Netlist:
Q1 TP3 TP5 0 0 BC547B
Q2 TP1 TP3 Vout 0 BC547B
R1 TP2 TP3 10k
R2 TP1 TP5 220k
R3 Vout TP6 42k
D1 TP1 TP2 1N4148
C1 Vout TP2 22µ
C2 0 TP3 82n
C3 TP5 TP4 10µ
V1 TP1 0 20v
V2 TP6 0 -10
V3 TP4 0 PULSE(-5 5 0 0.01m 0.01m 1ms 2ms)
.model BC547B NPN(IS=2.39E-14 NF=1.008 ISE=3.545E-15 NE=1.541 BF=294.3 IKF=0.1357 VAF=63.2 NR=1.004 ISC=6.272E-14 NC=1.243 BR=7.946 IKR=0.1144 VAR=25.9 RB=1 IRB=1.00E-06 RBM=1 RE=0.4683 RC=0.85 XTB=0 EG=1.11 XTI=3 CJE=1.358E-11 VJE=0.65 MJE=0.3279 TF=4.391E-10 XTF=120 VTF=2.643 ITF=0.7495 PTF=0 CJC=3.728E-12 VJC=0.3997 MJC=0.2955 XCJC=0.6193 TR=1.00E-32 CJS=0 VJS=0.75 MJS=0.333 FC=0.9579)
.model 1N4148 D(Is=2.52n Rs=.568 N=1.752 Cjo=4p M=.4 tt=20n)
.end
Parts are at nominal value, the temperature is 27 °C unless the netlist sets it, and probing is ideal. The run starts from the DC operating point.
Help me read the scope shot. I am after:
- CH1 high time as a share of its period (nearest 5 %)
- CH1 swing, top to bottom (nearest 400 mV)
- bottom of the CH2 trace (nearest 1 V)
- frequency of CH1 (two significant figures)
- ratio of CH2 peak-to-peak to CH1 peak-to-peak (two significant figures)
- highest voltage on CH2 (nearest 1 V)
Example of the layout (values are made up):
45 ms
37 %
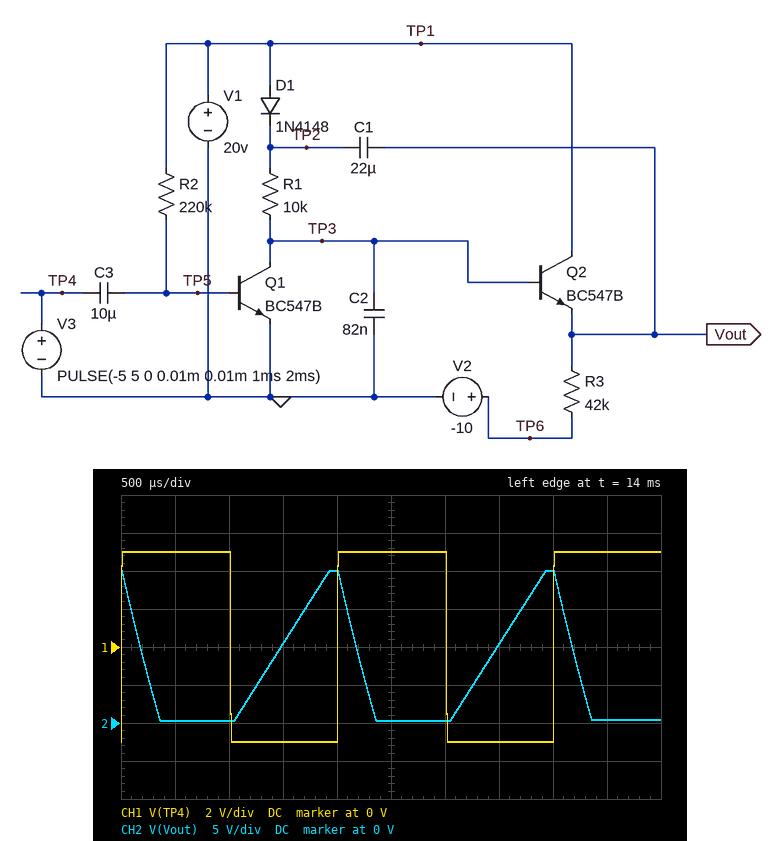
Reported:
50 %
10.0 V
0 V
500 Hz
2.0
20 V
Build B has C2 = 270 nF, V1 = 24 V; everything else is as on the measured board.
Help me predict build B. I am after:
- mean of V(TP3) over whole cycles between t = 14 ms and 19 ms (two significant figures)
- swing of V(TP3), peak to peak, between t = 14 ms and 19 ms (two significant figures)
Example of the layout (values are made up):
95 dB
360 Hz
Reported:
3.0 V
8.3 V
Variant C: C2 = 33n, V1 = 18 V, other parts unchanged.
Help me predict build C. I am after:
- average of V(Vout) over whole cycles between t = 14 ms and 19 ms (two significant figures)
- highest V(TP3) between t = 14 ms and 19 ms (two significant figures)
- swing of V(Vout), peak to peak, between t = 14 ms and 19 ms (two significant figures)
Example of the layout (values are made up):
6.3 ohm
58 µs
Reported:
8.1 V
19 V
18 V
